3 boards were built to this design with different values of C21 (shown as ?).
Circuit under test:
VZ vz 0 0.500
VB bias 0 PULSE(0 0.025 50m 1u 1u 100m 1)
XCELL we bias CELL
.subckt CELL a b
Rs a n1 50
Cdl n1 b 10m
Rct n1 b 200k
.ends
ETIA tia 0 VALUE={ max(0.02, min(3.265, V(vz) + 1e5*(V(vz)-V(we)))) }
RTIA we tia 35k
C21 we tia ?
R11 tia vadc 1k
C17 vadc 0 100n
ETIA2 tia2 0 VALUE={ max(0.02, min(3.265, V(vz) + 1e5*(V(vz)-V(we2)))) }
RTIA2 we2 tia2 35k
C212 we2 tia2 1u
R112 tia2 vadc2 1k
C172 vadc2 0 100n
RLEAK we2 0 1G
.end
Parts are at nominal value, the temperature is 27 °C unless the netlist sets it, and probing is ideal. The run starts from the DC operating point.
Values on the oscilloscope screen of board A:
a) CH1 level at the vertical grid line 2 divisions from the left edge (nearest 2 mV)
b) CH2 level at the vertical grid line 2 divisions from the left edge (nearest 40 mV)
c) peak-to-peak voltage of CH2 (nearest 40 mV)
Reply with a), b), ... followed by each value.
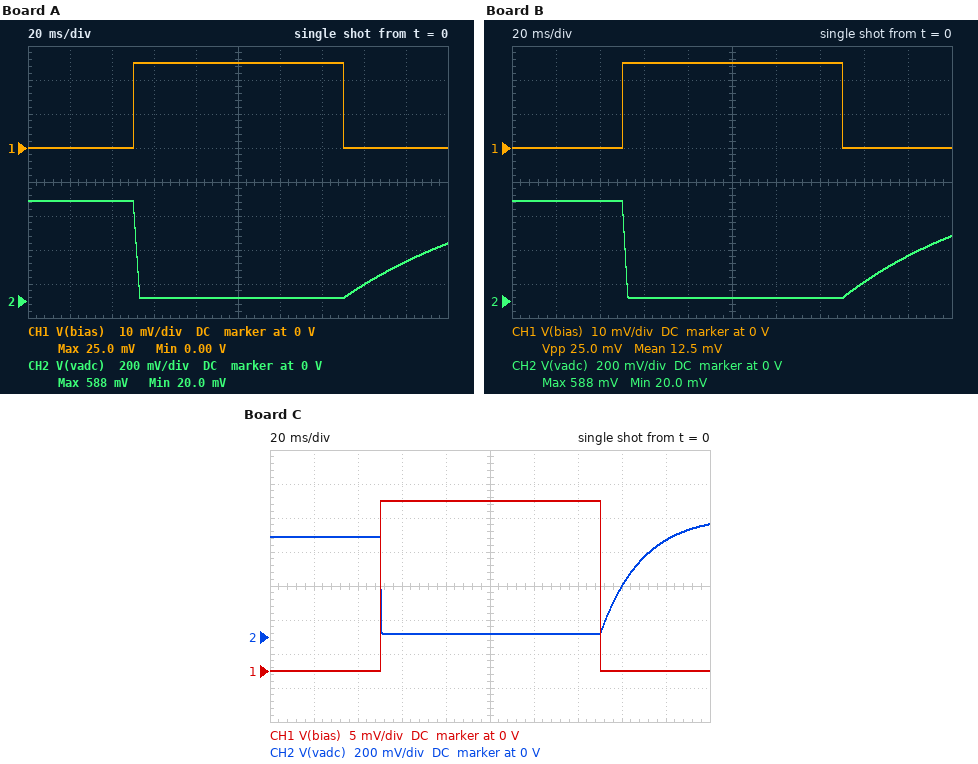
a) 0 V
b) 600 mV
c) 560 mV
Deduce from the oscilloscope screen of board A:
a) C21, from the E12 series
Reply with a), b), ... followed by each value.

a) 2.7 µF
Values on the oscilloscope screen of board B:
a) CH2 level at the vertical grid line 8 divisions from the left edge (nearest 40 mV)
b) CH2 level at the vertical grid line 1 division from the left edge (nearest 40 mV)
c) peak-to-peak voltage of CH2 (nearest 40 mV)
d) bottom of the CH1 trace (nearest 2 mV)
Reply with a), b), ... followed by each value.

a) 120 mV
b) 600 mV
c) 560 mV
d) 0 V
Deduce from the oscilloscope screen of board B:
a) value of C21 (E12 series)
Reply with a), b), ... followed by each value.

a) 2.2 µF
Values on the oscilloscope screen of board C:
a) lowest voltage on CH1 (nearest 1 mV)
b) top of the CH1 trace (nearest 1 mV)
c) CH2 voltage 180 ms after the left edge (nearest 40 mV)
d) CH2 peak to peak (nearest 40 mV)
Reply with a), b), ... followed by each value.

a) 0 V
b) 25 mV
c) 560 mV
d) 640 mV
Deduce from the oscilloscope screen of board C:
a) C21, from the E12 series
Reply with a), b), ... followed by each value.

a) 560 nF
